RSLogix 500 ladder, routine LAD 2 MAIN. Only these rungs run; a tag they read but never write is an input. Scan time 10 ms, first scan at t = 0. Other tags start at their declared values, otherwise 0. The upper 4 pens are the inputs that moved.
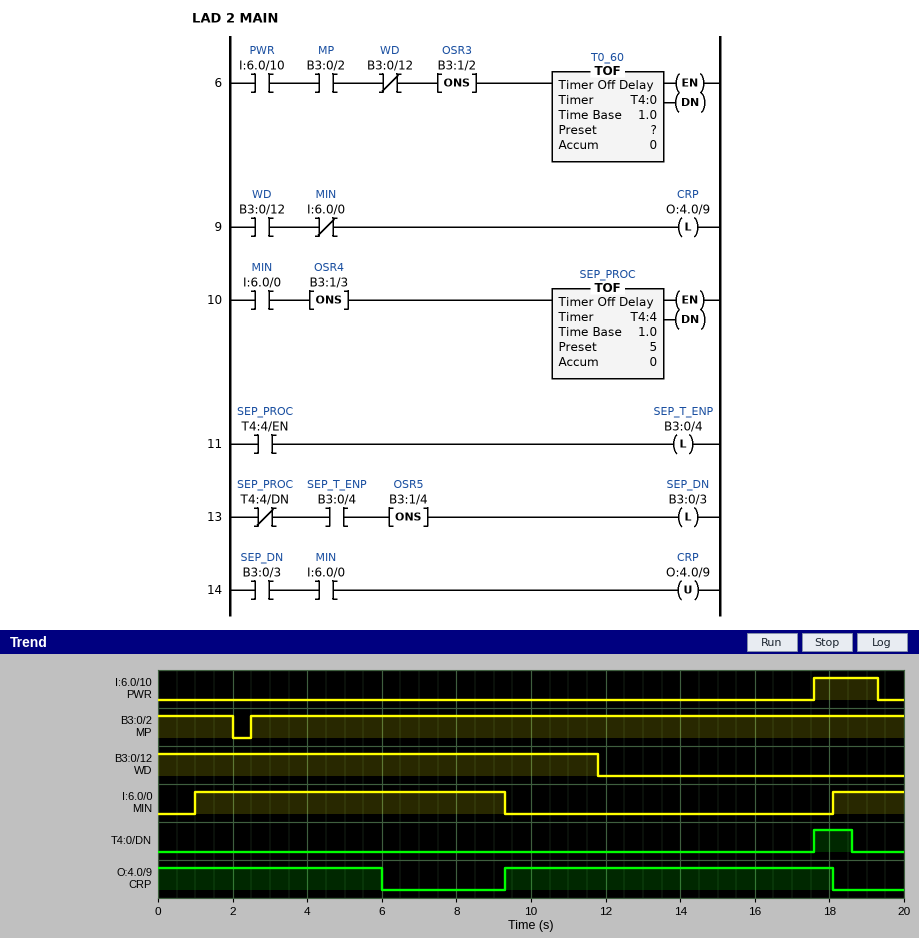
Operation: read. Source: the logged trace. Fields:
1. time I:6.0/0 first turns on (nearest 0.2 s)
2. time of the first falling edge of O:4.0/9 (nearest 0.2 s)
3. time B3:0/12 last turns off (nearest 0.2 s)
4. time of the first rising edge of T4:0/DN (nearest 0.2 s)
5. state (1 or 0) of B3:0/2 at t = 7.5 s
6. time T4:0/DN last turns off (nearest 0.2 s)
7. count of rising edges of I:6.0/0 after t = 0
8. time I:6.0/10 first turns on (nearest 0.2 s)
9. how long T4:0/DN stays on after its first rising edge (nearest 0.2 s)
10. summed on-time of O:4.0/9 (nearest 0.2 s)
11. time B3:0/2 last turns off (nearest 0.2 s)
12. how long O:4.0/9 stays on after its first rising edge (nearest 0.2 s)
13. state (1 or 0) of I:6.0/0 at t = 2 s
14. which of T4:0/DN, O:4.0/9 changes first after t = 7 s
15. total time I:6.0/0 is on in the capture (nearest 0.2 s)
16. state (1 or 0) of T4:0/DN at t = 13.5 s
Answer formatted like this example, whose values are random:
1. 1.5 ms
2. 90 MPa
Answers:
1. 1.0 s
2. 6.0 s
3. 11.8 s
4. 17.6 s
5. 1
6. 18.6 s
7. 2
8. 17.6 s
9. 1.0 s
10. 14.8 s
11. 2.0 s
12. 8.8 s
13. 1
14. O:4.0/9
15. 10.2 s
16. 0
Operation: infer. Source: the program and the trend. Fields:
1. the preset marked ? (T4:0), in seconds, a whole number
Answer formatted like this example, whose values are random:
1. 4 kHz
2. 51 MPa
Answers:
1. 1 s
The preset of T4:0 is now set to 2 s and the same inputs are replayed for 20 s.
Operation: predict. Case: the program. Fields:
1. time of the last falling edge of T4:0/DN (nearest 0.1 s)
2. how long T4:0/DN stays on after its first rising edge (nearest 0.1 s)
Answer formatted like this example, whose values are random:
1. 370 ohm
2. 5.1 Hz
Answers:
1. 19.6 s
2. 2.0 s
